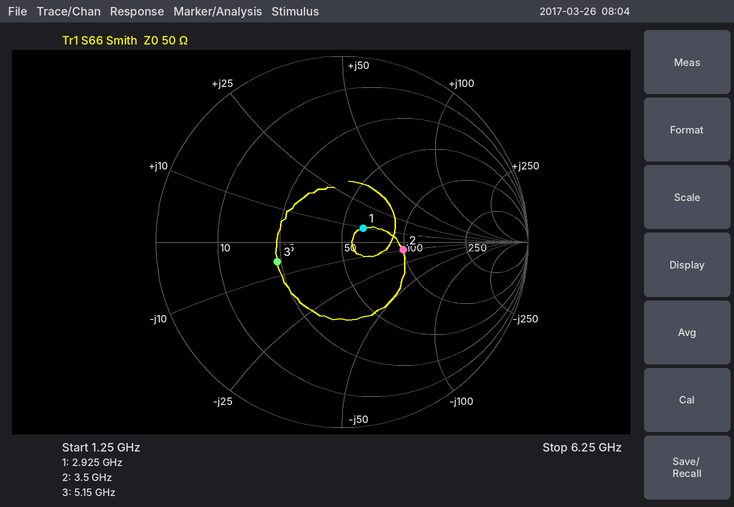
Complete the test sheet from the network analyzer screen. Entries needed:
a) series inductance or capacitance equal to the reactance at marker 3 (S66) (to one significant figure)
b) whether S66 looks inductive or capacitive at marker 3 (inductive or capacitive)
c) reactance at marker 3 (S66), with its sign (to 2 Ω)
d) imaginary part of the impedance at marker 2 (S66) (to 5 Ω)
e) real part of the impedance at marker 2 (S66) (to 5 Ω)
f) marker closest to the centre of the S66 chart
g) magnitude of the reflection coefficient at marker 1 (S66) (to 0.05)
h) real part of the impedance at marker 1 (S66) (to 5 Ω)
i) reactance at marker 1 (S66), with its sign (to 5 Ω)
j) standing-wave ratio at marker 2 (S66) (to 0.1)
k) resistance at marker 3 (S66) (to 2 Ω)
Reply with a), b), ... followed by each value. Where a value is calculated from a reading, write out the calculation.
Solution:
a) C = 1/(2π × 5.15 GHz × 6 Ω) ≈ 5 pF
b) capacitive
c) -6 Ω
d) -10 Ω
e) 100 Ω
f) marker 1
g) 0.15
h) 60 Ω
i) +10 Ω
j) 2.0
k) 24 Ω
